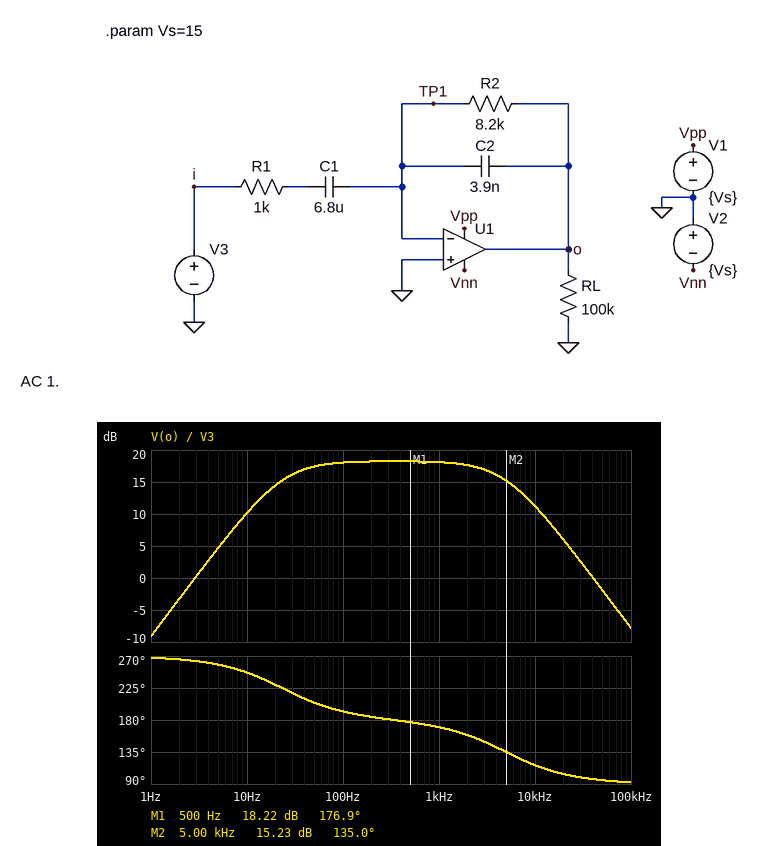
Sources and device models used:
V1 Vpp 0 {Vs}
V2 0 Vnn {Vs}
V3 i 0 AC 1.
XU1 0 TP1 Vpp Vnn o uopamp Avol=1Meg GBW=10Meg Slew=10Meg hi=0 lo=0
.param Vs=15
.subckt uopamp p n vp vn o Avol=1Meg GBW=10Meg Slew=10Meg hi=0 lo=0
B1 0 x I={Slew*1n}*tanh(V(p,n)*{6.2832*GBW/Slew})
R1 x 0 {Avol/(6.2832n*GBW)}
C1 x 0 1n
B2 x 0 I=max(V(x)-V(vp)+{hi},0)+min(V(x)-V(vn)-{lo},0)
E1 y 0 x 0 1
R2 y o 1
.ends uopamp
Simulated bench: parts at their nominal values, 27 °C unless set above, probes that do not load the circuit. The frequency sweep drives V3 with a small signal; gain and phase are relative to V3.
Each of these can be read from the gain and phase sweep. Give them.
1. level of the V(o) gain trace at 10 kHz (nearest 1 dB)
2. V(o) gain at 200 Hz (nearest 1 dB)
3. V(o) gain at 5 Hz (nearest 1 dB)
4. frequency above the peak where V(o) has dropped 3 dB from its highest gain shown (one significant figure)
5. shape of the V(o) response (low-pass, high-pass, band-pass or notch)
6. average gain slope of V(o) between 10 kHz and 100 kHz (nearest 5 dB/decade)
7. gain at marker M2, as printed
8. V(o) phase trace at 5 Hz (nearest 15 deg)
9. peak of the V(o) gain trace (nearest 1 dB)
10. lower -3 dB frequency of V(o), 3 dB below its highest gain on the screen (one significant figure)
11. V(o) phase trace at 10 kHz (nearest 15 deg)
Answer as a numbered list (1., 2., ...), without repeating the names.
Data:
1. 11 dB
2. 18 dB
3. 5 dB
4. 5 kHz
5. band-pass
6. -20 dB/decade
7. 15.23 dB
8. 255 deg
9. 18 dB
10. 20 Hz
11. 120 deg
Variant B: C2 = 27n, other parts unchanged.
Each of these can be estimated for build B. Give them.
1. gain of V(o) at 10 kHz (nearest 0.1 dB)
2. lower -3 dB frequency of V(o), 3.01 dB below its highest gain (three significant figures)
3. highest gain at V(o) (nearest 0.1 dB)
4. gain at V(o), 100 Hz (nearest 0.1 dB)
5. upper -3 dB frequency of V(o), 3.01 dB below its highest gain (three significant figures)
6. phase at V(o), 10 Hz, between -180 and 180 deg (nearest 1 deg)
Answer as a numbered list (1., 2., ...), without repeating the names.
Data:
1. -4.6 dB
2. 22.0 Hz
3. 18.0 dB
4. 18.0 dB
5. 764 Hz
6. -114 deg
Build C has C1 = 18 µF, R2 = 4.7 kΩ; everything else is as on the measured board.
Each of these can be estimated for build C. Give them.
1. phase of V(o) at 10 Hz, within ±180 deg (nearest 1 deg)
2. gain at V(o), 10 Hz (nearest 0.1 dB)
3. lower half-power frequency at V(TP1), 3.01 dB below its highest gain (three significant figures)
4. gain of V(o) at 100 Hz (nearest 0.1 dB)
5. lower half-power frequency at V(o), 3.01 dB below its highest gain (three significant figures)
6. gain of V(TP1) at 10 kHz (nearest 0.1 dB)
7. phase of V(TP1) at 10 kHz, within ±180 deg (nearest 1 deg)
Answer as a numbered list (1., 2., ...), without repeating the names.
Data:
1. -139 deg
2. 10.9 dB
3. 8.63 kHz
4. 13.4 dB
5. 8.82 Hz
6. -50.2 dB
7. 41 deg
